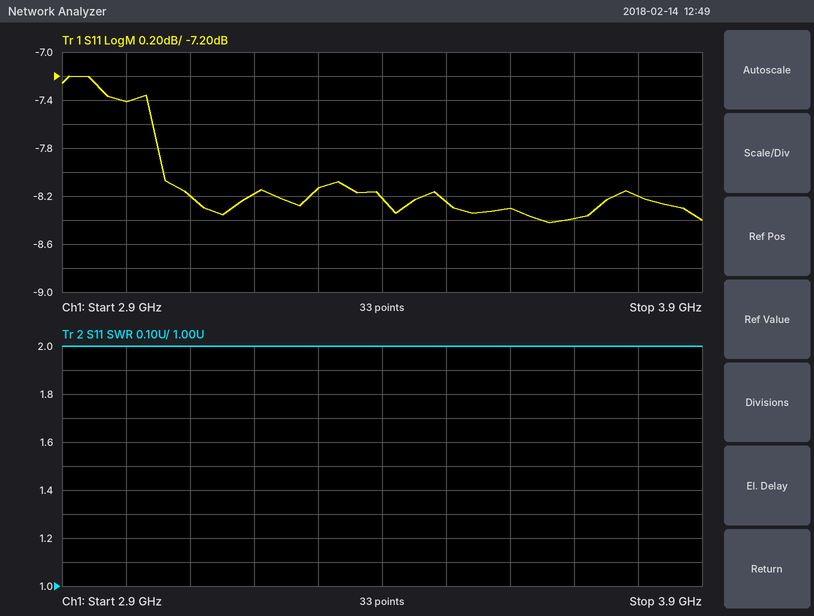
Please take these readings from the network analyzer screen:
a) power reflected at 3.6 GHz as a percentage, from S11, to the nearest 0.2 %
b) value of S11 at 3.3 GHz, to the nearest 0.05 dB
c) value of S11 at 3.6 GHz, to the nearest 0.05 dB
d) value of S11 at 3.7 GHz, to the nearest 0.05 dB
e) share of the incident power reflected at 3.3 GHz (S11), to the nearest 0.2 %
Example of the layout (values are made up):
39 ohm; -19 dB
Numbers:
14.8 %; -8.15 dB; -8.30 dB; -8.40 dB; 15.4 %
